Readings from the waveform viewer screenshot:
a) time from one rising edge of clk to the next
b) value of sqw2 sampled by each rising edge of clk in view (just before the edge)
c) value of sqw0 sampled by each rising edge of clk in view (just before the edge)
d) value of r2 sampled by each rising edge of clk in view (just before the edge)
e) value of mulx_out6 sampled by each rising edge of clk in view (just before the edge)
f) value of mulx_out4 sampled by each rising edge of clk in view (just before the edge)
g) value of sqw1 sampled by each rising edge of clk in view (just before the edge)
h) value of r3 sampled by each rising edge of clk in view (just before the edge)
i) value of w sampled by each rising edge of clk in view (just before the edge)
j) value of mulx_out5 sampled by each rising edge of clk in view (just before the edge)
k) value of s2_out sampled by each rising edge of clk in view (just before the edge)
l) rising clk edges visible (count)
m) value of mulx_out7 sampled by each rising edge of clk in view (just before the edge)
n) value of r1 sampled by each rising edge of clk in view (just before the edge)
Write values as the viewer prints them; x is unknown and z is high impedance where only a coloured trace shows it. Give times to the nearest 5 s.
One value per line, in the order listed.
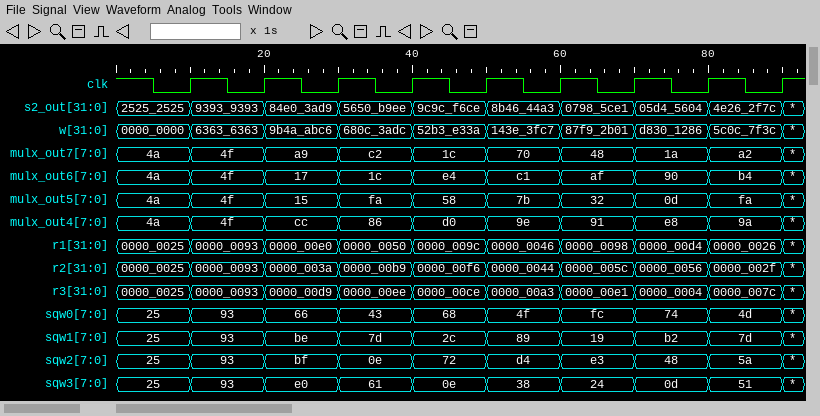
10 s
25, 93, bf, 0e, 72, d4, e3, 48, 5a
25, 93, 66, 43, 68, 4f, fc, 74, 4d
0000_0025, 0000_0093, 0000_003a, 0000_00b9, 0000_00f6, 0000_0044, 0000_005c, 0000_0056, 0000_002f
4a, 4f, 17, 1c, e4, c1, af, 90, b4
4a, 4f, cc, 86, d0, 9e, 91, e8, 9a
25, 93, be, 7d, 2c, 89, 19, b2, 7d
0000_0025, 0000_0093, 0000_00d9, 0000_00ee, 0000_00ce, 0000_00a3, 0000_00e1, 0000_0004, 0000_007c
0000_0000, 6363_6363, 9b4a_abc6, 680c_3adc, 52b3_e33a, 143e_3fc7, 87f9_2b01, d830_1286, 5c0c_7f3c
4a, 4f, 15, fa, 58, 7b, 32, 0d, fa
2525_2525, 9393_9393, 84e0_3ad9, 5650_b9ee, 9c9c_f6ce, 8b46_44a3, 0798_5ce1, 05d4_5604, 4e26_2f7c
9
4a, 4f, a9, c2, 1c, 70, 48, 1a, a2
0000_0025, 0000_0093, 0000_00e0, 0000_0050, 0000_009c, 0000_0046, 0000_0098, 0000_00d4, 0000_0026
